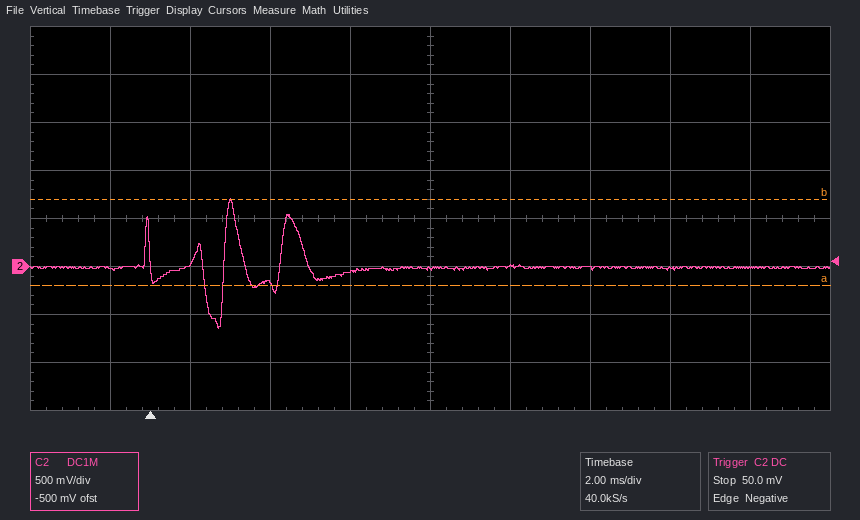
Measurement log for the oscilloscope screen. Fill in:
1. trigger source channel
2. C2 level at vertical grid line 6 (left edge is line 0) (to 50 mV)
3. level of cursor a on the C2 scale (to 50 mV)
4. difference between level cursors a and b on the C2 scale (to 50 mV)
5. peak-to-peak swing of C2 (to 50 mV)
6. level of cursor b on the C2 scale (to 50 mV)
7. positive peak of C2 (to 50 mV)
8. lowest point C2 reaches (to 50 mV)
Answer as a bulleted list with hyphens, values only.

- C2
- 0 mV
- -200 mV
- 900 mV
- 1.35 V
- 700 mV
- 700 mV
- -650 mV
